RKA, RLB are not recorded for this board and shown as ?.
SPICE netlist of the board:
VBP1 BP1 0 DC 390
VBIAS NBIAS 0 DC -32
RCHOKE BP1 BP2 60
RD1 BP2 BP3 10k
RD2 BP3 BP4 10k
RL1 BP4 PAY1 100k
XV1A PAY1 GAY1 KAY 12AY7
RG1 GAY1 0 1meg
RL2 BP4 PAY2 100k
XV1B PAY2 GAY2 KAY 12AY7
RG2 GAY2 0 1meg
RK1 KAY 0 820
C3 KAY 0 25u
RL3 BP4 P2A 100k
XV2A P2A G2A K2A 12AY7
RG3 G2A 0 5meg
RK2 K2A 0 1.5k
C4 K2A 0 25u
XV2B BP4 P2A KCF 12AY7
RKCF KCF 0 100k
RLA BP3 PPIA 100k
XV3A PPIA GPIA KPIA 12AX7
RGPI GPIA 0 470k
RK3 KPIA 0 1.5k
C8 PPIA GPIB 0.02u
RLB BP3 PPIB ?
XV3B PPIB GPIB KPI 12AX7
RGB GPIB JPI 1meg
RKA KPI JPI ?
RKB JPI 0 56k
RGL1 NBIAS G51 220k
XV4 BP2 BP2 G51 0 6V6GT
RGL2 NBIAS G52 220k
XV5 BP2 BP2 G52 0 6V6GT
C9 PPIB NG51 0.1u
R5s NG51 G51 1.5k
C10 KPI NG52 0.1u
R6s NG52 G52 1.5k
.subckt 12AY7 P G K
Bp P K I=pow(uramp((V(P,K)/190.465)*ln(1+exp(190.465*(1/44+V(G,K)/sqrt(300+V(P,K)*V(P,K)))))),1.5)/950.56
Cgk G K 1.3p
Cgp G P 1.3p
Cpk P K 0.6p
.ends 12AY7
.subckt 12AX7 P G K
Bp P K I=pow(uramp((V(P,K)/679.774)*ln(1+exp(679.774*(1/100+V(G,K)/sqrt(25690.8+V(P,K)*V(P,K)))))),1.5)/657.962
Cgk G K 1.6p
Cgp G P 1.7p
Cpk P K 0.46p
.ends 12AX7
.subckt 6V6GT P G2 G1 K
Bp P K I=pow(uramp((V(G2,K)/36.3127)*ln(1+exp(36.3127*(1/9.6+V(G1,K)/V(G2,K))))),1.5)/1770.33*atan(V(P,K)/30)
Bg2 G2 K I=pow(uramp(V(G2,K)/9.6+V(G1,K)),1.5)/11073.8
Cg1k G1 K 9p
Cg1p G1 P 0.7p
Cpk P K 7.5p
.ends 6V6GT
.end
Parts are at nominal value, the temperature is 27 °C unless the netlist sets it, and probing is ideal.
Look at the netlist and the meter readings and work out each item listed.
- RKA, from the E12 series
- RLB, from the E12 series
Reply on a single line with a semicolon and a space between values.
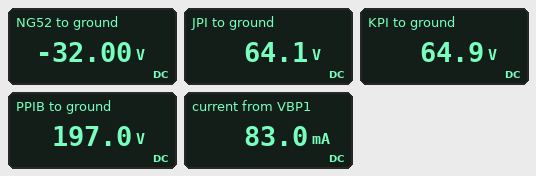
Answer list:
680 Ω; 100 kΩ
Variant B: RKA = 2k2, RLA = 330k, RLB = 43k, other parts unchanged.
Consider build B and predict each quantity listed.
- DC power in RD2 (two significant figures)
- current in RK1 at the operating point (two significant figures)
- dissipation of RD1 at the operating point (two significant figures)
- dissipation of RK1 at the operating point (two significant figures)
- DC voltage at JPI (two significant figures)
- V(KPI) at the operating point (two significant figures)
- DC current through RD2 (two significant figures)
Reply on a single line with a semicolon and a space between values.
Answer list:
270 mW; 2.6 mA; 460 mW; 5.4 mW; 50 V; 52 V; 5.2 mA
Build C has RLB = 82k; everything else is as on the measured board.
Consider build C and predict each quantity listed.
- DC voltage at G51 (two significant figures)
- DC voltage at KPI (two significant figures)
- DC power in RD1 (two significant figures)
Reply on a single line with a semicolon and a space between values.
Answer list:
-32 V; 69 V; 550 mW
